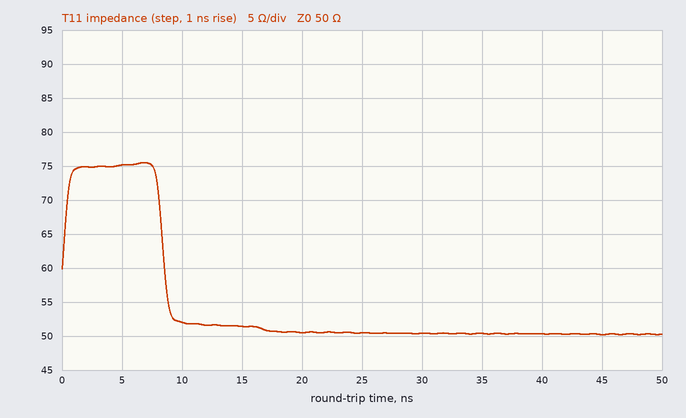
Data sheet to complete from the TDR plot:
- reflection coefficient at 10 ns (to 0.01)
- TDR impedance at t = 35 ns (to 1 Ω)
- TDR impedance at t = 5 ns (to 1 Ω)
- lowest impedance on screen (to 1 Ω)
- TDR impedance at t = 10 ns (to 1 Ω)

+0.02
50 Ω
75 Ω
50 Ω
52 Ω
